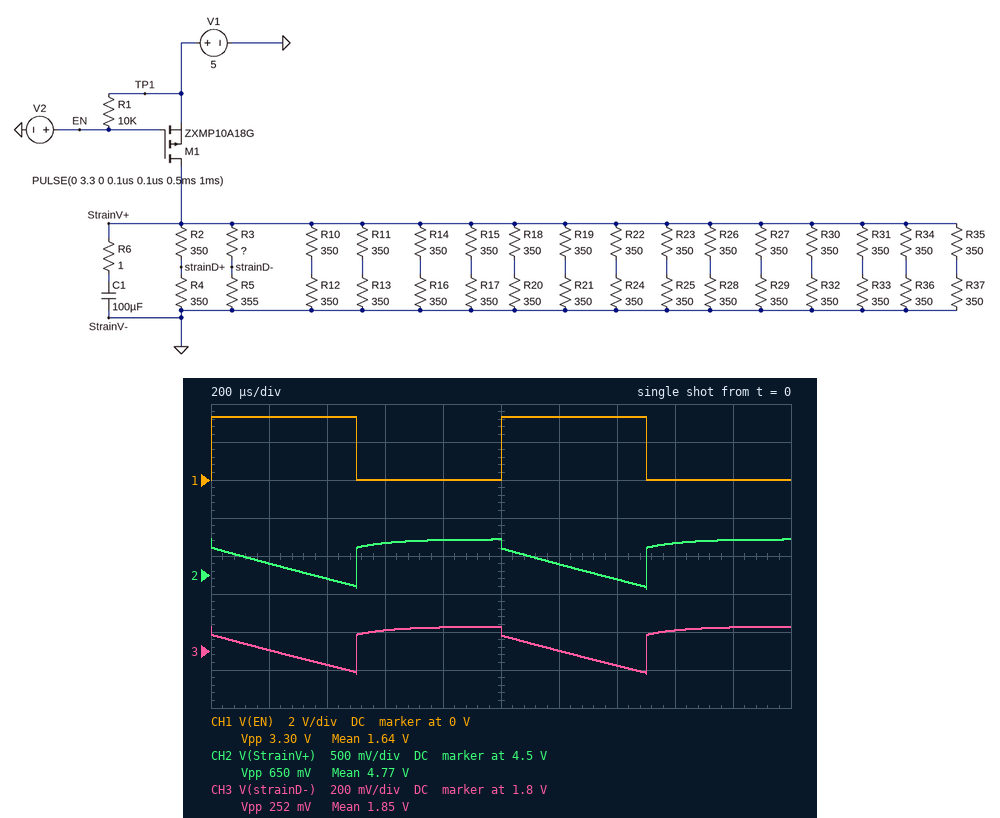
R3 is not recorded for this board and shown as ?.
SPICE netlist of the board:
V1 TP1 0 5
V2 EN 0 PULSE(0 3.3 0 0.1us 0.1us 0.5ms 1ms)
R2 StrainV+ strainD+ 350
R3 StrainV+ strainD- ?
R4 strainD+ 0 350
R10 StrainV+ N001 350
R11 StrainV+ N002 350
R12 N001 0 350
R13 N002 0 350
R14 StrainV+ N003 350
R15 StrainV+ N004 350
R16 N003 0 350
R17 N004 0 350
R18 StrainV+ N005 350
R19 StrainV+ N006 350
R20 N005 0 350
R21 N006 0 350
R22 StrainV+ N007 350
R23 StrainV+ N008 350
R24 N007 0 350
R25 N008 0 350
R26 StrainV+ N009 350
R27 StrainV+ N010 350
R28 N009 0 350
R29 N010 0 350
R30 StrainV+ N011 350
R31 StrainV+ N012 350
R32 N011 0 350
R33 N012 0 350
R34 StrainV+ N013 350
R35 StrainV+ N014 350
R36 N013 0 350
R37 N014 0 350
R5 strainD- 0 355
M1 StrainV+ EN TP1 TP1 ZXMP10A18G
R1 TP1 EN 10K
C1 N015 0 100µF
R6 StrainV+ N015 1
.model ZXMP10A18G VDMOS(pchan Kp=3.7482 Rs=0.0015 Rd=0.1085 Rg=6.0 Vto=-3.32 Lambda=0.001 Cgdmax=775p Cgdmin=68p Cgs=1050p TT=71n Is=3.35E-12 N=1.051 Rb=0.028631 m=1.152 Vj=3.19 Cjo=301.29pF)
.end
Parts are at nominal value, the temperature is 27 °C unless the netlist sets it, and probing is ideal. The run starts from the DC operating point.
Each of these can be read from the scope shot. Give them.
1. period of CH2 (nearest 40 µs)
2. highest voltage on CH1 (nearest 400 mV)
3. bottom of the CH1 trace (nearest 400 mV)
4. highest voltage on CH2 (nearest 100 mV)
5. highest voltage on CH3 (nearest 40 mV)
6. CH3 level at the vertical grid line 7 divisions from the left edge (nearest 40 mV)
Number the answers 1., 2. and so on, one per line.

1. 1.00 ms
2. 3.2 V
3. 0 V
4. 5.0 V
5. 1.92 V
6. 1.72 V
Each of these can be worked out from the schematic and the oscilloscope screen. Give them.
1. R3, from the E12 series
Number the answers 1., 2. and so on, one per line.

1. 560 Ω
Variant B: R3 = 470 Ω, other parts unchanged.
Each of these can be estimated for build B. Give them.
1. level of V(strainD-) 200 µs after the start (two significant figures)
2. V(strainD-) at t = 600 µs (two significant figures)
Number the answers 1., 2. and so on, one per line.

1. 2.0 V
2. 2.1 V
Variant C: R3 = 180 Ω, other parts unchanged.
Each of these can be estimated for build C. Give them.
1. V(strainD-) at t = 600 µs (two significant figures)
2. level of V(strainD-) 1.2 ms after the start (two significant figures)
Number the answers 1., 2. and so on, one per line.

1. 3.3 V
2. 3.1 V
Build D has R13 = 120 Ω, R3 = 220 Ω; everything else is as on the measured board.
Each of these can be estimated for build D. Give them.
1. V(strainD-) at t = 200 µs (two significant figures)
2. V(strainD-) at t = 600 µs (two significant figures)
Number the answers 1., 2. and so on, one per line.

1. 2.9 V
2. 3.0 V
